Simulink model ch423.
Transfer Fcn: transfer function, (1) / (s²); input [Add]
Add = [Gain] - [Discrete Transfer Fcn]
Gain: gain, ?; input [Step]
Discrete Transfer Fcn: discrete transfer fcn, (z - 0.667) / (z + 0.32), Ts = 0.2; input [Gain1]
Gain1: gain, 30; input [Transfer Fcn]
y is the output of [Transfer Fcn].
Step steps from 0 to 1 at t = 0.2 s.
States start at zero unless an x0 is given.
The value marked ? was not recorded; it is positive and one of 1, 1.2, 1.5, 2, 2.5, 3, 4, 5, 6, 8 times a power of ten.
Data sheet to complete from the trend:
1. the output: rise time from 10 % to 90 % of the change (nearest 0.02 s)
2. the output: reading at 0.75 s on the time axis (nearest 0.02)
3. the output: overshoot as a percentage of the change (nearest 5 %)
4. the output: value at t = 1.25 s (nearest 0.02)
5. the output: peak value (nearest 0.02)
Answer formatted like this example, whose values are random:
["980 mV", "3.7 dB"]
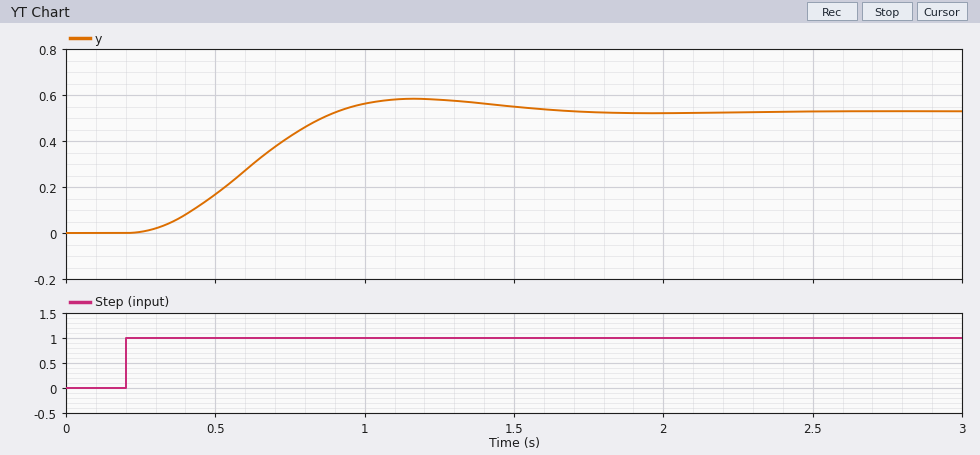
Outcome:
["0.46 s", "0.42", "10 %", "0.58", "0.58"]
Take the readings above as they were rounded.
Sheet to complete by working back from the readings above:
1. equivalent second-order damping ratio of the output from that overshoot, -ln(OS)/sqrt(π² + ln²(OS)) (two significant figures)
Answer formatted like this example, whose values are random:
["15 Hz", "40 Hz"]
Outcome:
["0.59"]
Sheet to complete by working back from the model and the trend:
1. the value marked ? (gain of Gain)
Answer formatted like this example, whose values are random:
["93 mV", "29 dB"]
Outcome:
["4"]
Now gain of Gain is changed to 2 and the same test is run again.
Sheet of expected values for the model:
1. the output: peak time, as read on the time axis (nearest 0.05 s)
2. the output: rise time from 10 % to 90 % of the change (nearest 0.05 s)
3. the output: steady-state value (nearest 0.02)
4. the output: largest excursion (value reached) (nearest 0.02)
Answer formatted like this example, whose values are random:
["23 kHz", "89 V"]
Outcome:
["1.15 s", "0.45 s", "0.26", "0.30"]
